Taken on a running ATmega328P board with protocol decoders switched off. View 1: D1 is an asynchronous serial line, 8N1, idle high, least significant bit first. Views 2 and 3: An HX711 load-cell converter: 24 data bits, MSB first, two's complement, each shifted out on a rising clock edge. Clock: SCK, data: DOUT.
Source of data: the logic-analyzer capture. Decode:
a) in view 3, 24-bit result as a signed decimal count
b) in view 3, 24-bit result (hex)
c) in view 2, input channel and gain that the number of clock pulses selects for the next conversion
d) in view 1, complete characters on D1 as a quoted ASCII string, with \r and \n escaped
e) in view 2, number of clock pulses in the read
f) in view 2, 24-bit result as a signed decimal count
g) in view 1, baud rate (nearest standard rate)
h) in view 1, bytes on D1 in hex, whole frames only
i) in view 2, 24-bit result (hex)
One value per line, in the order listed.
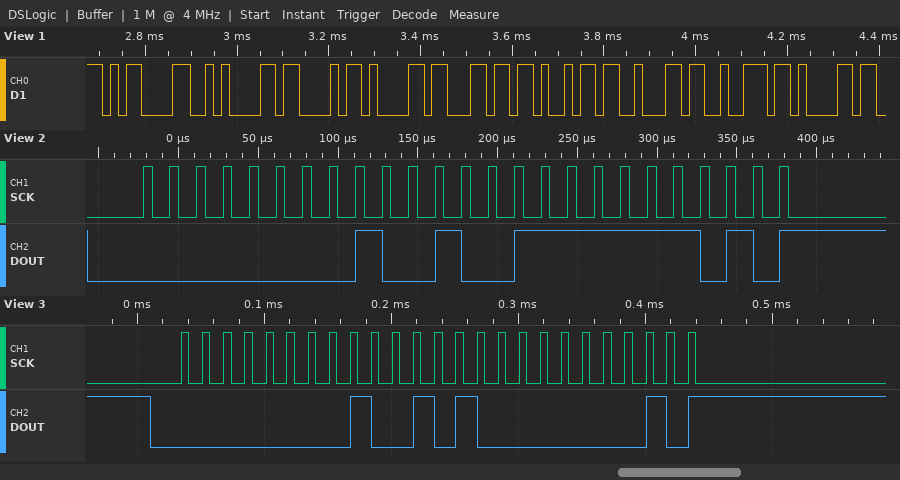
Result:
37890
0x009402
channel A, gain 128
"\r\nCalibra"
25
37882
57600 baud
0D 0A 43 61 6C 69 62 72 61
0x0093FA
